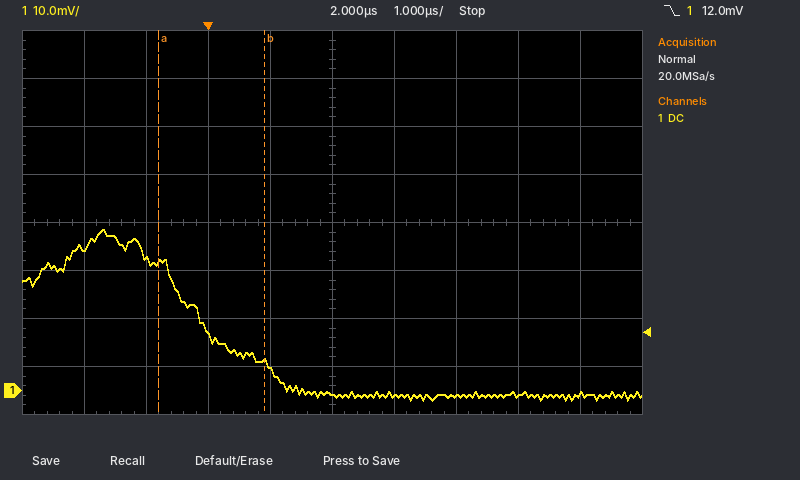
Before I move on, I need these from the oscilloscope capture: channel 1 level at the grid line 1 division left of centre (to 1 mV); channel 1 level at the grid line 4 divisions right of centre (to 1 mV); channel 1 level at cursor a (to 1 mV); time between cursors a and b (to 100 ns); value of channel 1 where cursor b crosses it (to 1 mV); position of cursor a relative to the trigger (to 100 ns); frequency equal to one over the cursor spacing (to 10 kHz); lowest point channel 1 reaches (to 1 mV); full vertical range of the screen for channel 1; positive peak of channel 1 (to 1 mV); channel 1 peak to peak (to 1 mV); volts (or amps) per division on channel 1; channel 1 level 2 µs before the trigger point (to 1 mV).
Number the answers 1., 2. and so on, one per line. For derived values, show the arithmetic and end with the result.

1. 5 mV
2. -1 mV
3. 27 mV
4. 1.7 µs
5. 6 mV
6. -800 ns
7. 1 / 1.7 µs ≈ 590 kHz
8. -2 mV
9. 80 mV
10. 34 mV
11. 34 mV − (-2 mV) = 36 mV
12. 10 mV
13. 30 mV
